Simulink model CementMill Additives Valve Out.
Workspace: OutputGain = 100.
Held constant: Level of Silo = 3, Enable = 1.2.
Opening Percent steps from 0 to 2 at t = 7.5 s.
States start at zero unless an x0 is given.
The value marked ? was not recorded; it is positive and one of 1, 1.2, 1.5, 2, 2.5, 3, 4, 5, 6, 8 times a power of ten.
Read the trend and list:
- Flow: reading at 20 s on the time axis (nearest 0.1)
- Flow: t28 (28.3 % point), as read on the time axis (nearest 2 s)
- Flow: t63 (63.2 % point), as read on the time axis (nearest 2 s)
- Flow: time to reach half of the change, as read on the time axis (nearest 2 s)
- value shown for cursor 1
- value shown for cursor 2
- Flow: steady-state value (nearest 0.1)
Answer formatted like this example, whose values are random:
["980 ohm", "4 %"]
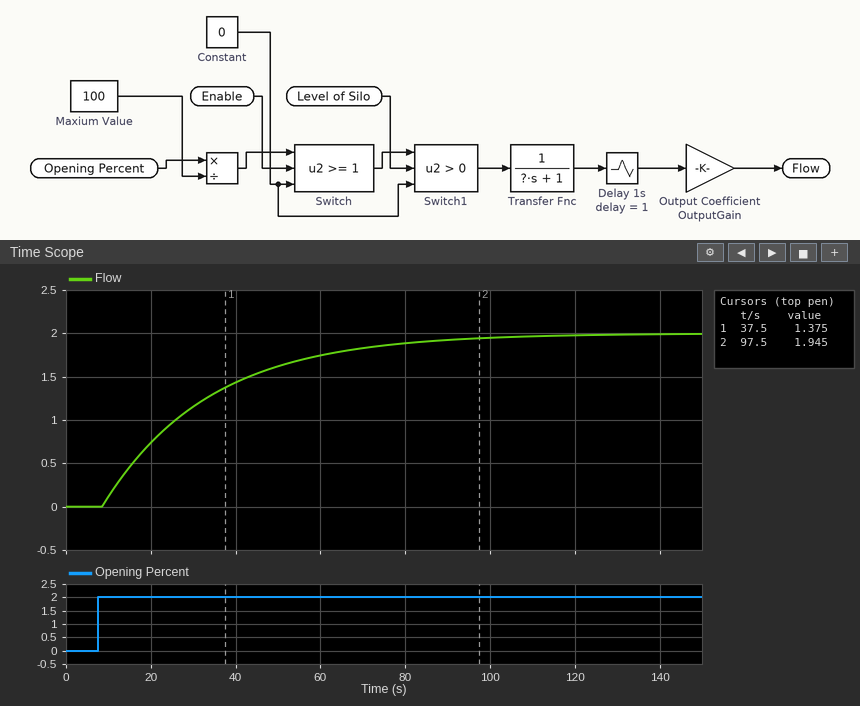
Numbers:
["0.7", "16 s", "34 s", "26 s", "1.375", "1.945", "2.0"]
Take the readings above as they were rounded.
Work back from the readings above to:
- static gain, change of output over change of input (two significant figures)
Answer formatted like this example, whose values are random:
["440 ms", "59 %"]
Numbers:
["1.0"]
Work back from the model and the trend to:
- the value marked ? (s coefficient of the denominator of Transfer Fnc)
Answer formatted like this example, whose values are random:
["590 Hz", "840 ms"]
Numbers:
["25"]
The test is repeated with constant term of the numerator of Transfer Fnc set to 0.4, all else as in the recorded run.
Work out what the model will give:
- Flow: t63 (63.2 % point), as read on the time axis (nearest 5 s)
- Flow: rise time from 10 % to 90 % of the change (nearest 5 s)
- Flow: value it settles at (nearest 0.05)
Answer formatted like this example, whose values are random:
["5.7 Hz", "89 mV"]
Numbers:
["35 s", "55 s", "0.80"]
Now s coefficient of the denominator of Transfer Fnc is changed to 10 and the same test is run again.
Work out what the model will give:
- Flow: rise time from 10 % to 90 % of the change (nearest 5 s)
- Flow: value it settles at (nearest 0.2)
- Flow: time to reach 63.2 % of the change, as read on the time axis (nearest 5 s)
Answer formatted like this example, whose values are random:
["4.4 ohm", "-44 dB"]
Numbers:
["20 s", "2.0", "20 s"]
